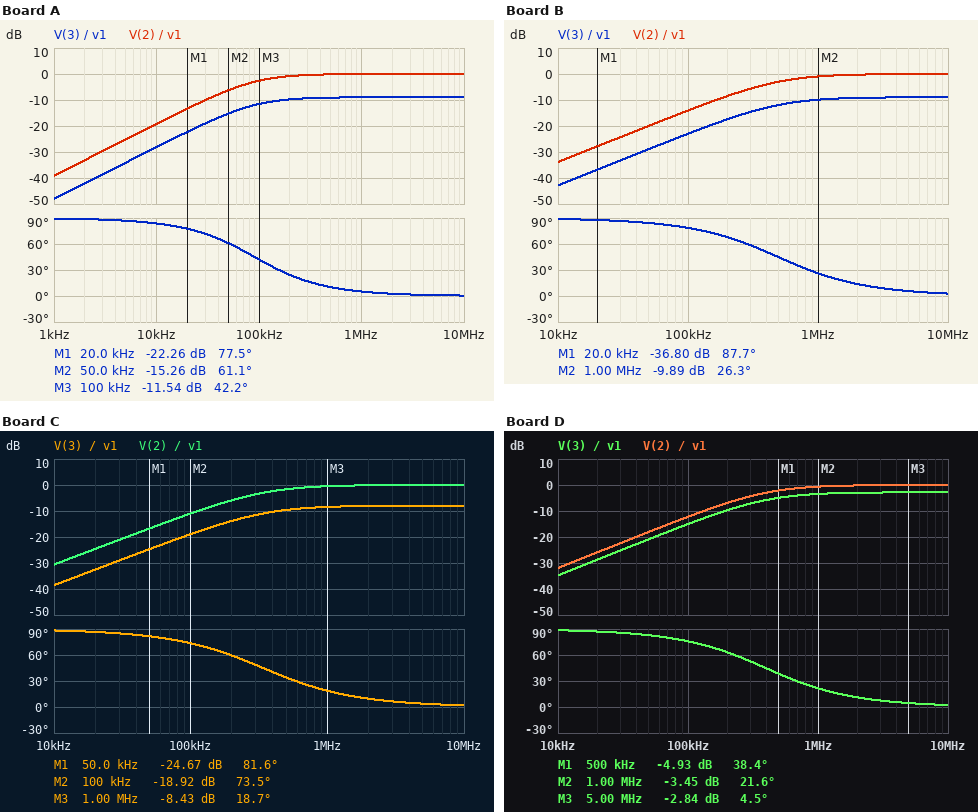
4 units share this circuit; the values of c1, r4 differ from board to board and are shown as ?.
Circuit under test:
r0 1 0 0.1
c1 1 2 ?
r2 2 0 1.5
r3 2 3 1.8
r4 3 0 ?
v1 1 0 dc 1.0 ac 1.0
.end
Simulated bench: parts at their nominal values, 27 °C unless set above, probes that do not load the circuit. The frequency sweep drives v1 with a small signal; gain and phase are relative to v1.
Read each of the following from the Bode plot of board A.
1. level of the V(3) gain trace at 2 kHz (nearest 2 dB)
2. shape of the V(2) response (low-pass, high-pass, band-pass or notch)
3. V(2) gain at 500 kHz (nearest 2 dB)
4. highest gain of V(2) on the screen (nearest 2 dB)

-42 dB
high-pass
0 dB
0 dB
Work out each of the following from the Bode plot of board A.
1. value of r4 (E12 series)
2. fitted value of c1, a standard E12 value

1 Ω
1.8 µF
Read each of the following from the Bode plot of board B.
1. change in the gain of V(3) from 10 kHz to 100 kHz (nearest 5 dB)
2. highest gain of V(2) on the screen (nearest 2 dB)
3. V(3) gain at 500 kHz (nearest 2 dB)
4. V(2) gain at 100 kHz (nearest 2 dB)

20 dB
0 dB
-12 dB
-14 dB
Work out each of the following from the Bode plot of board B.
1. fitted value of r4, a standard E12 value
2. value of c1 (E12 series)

1 Ω
330 nF
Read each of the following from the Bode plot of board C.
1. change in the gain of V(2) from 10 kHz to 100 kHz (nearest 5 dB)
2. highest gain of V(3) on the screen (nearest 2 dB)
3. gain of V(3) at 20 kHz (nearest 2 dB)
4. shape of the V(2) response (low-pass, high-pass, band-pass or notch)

20 dB
-8 dB
-32 dB
high-pass
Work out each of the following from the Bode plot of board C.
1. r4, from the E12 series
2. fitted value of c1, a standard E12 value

1.2 Ω
470 nF
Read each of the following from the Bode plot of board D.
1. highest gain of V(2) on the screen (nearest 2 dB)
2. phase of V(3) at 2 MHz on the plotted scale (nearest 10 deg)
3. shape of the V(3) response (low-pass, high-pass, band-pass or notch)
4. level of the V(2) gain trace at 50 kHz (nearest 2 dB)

0 dB
10 deg
high-pass
-18 dB
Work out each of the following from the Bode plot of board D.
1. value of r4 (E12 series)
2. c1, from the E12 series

4.7 Ω
330 nF
